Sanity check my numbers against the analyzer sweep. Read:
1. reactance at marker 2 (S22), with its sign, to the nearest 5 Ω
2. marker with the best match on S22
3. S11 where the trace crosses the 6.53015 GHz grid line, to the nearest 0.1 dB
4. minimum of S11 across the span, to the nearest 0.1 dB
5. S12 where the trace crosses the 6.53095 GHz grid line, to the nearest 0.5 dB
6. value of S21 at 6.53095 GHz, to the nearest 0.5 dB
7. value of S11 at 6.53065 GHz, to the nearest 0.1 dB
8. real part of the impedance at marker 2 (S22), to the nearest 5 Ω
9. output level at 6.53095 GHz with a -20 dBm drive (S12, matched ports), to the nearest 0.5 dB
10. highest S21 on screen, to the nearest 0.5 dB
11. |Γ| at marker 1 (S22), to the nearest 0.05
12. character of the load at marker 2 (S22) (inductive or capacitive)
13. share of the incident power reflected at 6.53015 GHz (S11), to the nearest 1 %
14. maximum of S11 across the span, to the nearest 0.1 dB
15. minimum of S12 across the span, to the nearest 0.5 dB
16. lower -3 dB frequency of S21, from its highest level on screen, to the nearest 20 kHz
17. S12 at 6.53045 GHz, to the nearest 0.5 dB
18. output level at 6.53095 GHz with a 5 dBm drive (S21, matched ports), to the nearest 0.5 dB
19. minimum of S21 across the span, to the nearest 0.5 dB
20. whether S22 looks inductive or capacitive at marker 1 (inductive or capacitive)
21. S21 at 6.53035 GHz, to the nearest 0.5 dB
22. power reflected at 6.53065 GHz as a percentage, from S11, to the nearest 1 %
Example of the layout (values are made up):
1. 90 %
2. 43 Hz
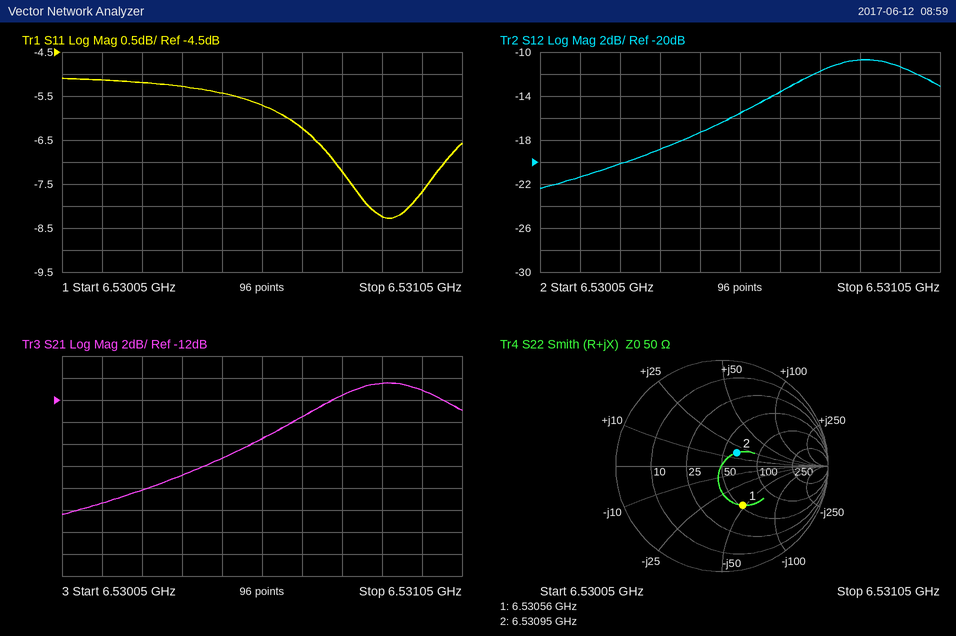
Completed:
1. +15 Ω
2. marker 2
3. -5.1 dB
4. -8.3 dB
5. -11.5 dB
6. -11.0 dB
7. -6.2 dB
8. 65 Ω
9. -31.5 dBm
10. -10.5 dB
11. 0.40
12. inductive
13. 31 %
14. -5.1 dB
15. -22.5 dB
16. 6.53066 GHz
17. -17.5 dB
18. -6.0 dBm
19. -22.5 dB
20. capacitive
21. -19.0 dB
22. 24 %
